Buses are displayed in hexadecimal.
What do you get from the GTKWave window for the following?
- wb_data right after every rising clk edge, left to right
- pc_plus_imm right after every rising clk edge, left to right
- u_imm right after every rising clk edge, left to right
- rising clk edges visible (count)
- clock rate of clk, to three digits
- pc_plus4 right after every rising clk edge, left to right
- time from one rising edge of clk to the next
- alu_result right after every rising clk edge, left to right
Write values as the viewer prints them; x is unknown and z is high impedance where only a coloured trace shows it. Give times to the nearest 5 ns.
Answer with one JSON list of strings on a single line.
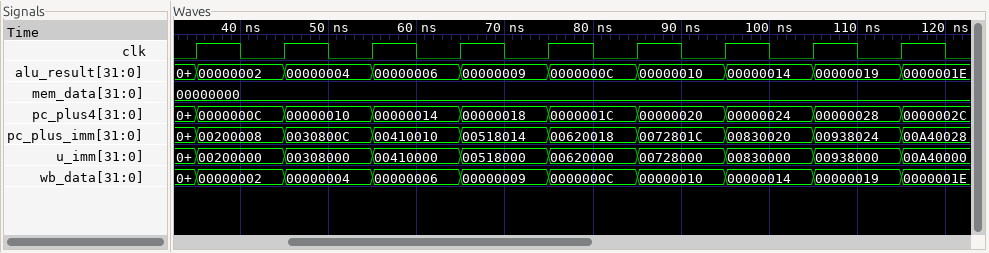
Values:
["00000002, 00000004, 00000006, 00000009, 0000000C, 00000010, 00000014, 00000019, 0000001E", "00200008, 0030800C, 00410010, 00518014, 00620018, 0072801C, 00830020, 00938024, 00A40028", "00200000, 00308000, 00410000, 00518000, 00620000, 00728000, 00830000, 00938000, 00A40000", "9", "100 MHz", "0000000C, 00000010, 00000014, 00000018, 0000001C, 00000020, 00000024, 00000028, 0000002C", "10 ns", "00000002, 00000004, 00000006, 00000009, 0000000C, 00000010, 00000014, 00000019, 0000001E"]
